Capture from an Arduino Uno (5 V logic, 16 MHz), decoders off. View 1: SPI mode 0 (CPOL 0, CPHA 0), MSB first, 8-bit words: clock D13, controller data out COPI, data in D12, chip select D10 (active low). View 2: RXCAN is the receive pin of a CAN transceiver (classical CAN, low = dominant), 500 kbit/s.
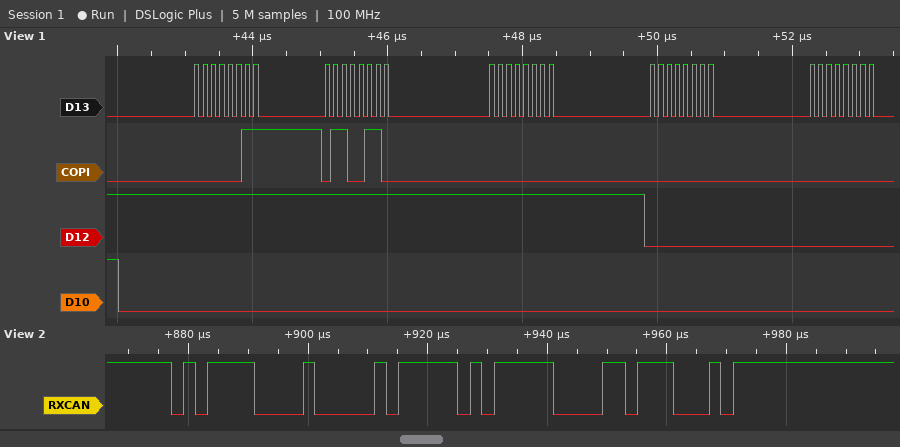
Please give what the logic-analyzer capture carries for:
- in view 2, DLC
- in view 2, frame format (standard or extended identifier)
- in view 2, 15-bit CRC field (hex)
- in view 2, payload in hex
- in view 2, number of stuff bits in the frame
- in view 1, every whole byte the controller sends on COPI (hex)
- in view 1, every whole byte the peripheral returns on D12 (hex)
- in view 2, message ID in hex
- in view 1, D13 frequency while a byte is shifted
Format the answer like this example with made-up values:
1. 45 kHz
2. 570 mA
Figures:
1. 1
2. standard
3. 0x71B8
4. FB
5. 3
6. 0x03 0x66 0x00 0x00 0x00
7. 0xFF 0xFF 0xFF 0x00 0x00
8. 0x5E1
9. 8 MHz
